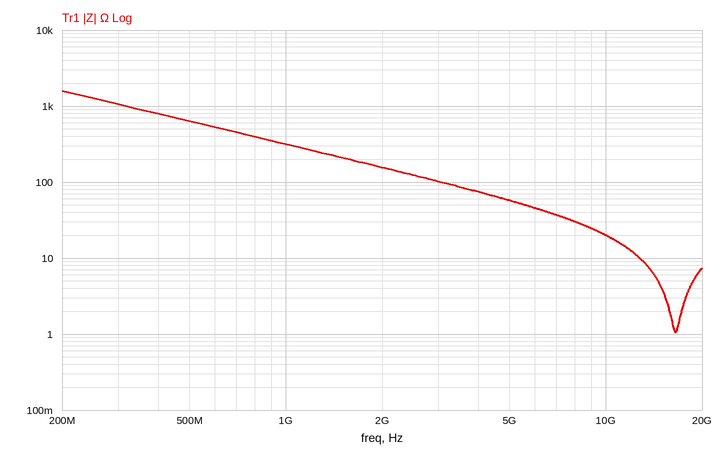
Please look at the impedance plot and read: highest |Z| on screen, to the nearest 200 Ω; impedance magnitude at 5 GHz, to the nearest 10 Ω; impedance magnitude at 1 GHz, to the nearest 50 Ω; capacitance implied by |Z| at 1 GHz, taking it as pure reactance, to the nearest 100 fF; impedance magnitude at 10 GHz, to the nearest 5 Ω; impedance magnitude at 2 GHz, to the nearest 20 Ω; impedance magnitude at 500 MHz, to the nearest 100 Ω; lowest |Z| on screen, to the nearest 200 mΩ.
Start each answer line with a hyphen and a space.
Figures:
- 1.6 kΩ
- 60 Ω
- 300 Ω
- 500 fF
- 20 Ω
- 160 Ω
- 600 Ω
- 1.0 Ω
